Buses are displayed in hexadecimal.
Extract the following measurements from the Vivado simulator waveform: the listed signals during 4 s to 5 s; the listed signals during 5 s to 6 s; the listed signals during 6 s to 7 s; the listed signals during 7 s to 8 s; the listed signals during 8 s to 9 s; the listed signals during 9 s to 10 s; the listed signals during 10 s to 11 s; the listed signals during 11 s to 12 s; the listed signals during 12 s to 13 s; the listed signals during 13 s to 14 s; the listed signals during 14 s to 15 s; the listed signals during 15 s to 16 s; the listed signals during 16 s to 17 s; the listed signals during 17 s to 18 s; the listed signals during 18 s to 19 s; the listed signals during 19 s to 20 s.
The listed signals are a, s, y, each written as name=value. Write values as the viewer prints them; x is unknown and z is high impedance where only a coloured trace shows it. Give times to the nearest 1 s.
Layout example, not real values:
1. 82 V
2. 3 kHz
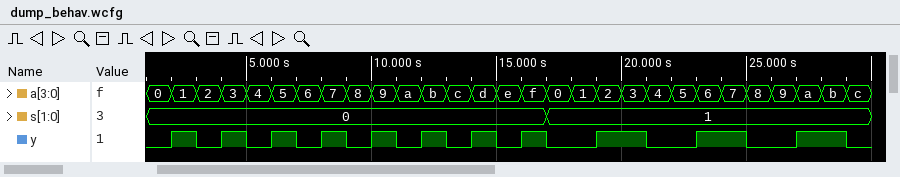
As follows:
1. a=3, s=0, y=1
2. a=4, s=0, y=0
3. a=5, s=0, y=1
4. a=6, s=0, y=0
5. a=7, s=0, y=1
6. a=8, s=0, y=0
7. a=9, s=0, y=1
8. a=a, s=0, y=0
9. a=b, s=0, y=1
10. a=c, s=0, y=0
11. a=d, s=0, y=1
12. a=e, s=0, y=0
13. a=f, s=0, y=1
14. a=0, s=1, y=0
15. a=1, s=1, y=0
16. a=2, s=1, y=1
